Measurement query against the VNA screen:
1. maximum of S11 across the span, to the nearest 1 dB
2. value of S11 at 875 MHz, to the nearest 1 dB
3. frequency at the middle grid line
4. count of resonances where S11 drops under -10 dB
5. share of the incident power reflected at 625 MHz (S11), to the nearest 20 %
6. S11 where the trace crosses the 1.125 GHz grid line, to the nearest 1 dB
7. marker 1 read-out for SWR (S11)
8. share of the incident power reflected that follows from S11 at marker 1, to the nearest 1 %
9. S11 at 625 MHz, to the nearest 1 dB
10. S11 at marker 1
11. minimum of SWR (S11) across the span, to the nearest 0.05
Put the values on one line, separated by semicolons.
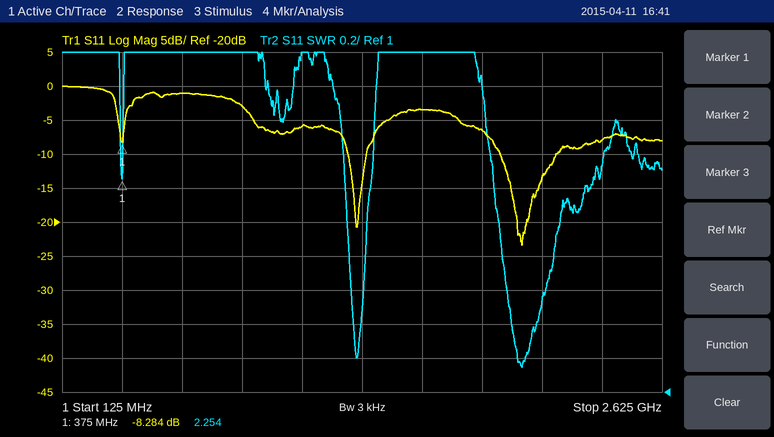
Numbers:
0 dB; -3 dB; 1.375 GHz; 2; 80 %; -6 dB; 2.254; 15 %; -1 dB; -8.284 dB; 1.15
